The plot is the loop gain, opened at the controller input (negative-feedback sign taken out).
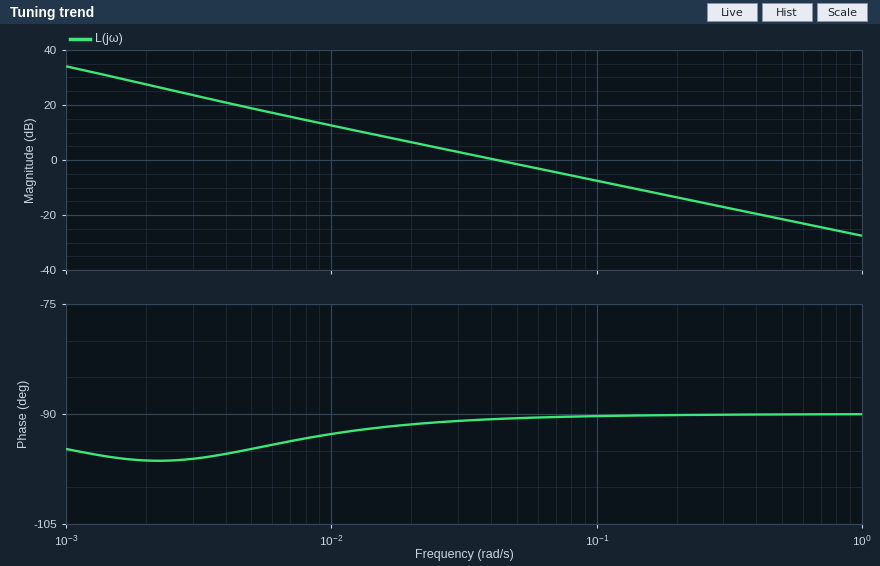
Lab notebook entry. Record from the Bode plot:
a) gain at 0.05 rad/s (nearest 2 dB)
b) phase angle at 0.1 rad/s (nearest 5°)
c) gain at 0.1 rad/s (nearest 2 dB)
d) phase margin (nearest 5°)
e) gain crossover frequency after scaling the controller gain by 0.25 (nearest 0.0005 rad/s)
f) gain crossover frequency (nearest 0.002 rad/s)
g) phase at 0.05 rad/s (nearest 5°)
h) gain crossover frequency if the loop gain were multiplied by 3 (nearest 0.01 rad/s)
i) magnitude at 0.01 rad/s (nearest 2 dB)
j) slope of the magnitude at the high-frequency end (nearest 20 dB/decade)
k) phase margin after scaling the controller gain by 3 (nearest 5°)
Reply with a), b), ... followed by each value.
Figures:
a) -2 dB
b) -90°
c) -8 dB
d) 90°
e) 0.0105 rad/s
f) 0.042 rad/s
g) -90°
h) 0.13 rad/s
i) 12 dB
j) -20 dB/decade
k) 90°
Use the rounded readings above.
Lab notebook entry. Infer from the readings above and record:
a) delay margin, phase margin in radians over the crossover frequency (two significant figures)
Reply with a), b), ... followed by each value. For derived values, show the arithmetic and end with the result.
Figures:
a) 90 × π / 180 / 0.042 = 37 s
